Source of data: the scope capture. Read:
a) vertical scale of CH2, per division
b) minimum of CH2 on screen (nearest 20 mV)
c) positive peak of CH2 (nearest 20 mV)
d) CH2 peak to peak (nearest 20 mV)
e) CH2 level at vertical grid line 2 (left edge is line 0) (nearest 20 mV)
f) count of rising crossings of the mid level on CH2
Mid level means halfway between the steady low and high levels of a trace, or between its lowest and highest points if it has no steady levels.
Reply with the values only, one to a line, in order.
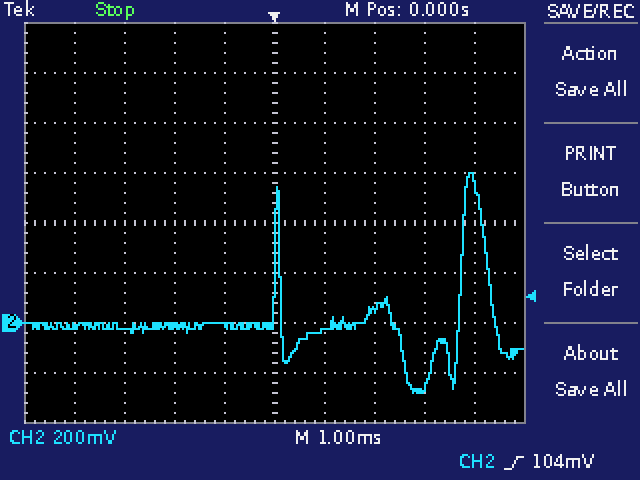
200 mV
-280 mV
600 mV
880 mV
-20 mV
2
